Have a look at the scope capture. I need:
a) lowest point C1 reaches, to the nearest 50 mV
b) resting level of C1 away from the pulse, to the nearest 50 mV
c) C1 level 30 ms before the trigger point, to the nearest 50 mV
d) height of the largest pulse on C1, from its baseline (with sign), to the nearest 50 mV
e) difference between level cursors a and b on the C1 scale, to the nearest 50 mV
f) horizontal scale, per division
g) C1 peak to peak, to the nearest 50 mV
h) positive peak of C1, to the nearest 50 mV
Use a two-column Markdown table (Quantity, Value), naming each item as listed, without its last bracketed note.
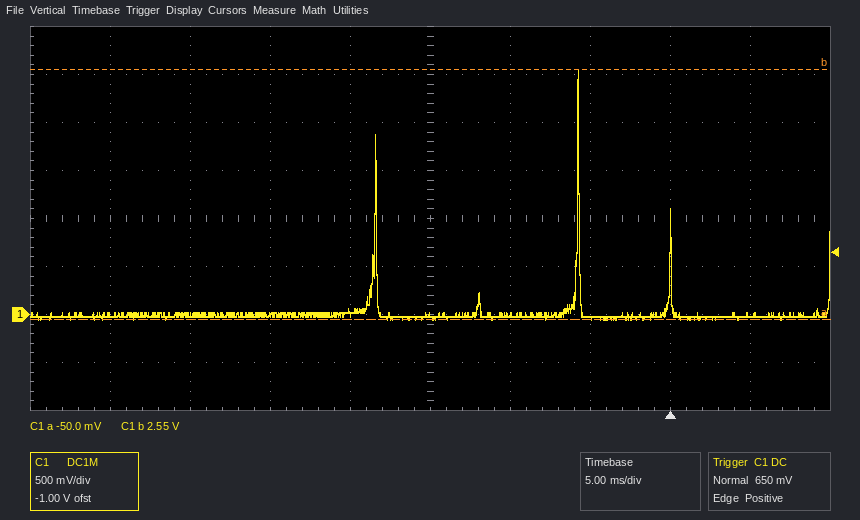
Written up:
| Quantity | Value |
|---|---|
| lowest point C1 reaches, to the nearest 50 mV | -50 mV |
| resting level of C1 away from the pulse, to the nearest 50 mV | 0 mV |
| C1 level 30 ms before the trigger point, to the nearest 50 mV | 0 mV |
| height of the largest pulse on C1, from its baseline (with sign), to the nearest 50 mV | +2.55 V |
| difference between level cursors a and b on the C1 scale, to the nearest 50 mV | 2.60 V |
| horizontal scale, per division | 5 ms |
| C1 peak to peak, to the nearest 50 mV | 2.60 V |
| positive peak of C1, to the nearest 50 mV | 2.55 V |
